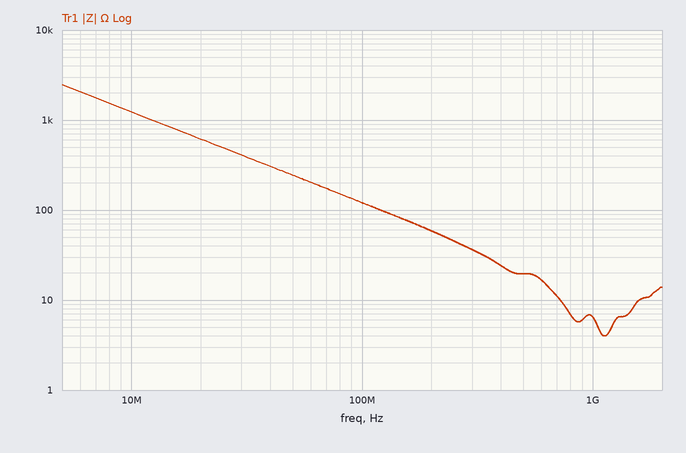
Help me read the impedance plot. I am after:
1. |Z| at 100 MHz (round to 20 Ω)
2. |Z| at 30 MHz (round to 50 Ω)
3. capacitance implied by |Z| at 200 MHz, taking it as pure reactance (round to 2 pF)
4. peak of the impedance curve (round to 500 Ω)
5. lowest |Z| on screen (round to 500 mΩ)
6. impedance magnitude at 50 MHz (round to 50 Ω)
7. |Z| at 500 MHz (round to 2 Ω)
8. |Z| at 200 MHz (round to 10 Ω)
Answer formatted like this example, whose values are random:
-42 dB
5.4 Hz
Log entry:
120 Ω
400 Ω
14 pF
2.5 kΩ
4.0 Ω
250 Ω
20 Ω
60 Ω
